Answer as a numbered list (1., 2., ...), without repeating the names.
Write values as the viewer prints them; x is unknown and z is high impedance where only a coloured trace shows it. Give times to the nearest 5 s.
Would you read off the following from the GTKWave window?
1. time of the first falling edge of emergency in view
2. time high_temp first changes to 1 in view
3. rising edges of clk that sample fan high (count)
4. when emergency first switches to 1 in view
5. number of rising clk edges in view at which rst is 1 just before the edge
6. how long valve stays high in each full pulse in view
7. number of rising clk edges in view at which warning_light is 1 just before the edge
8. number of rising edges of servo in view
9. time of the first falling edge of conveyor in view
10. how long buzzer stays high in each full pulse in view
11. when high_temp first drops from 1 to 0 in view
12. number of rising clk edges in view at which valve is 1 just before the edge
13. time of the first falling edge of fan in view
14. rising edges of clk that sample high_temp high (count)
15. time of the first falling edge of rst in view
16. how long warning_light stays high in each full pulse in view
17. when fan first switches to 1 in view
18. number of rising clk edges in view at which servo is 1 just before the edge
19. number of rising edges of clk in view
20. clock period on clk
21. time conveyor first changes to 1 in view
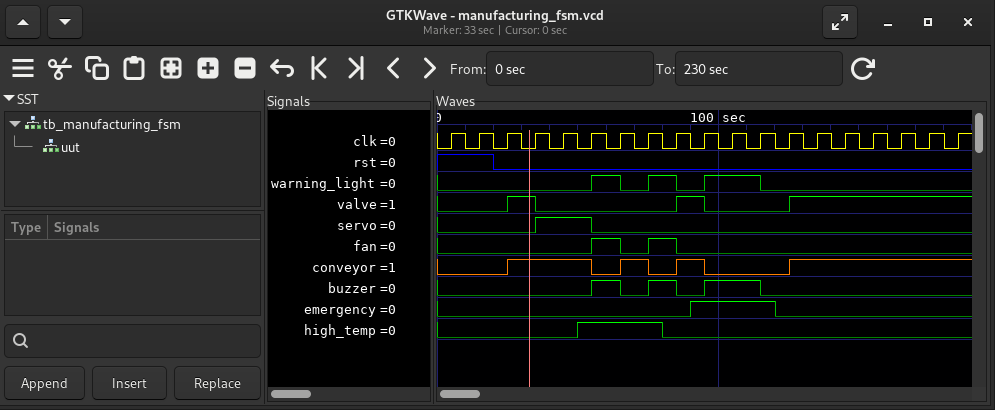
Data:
1. 120 s
2. 50 s
3. 2
4. 90 s
5. 2
6. 10 s, 10 s
7. 4
8. 1
9. 55 s
10. 10 s, 10 s, 20 s
11. 80 s
12. 8
13. 65 s
14. 3
15. 20 s
16. 10 s, 10 s, 20 s
17. 55 s
18. 2
19. 19
20. 10 s
21. 25 s
